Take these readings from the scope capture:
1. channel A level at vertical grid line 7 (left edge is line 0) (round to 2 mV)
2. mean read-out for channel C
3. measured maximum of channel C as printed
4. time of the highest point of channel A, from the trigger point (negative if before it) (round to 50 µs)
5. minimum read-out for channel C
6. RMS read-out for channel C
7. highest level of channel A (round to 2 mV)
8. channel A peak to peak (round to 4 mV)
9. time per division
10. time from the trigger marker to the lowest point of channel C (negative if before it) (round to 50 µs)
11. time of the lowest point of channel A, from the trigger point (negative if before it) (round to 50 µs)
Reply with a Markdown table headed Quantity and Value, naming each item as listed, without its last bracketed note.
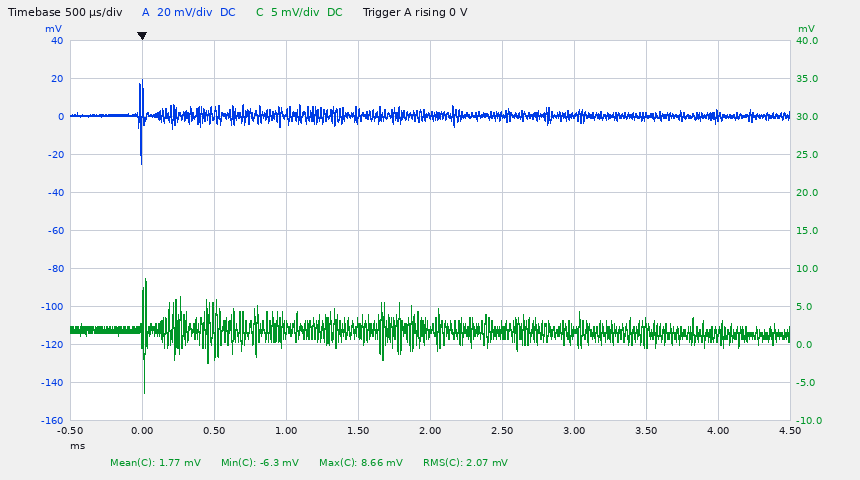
| Quantity | Value |
|---|---|
| channel A level at vertical grid line 7 (left edge is line 0) | 0 mV |
| mean read-out for channel C | 1.77 mV |
| measured maximum of channel C as printed | 8.66 mV |
| time of the highest point of channel A, from the trigger point (negative if before it) | 0 µs |
| minimum read-out for channel C | -6.3 mV |
| RMS read-out for channel C | 2.07 mV |
| highest level of channel A | 20 mV |
| channel A peak to peak | 44 mV |
| time per division | 500 µs |
| time from the trigger marker to the lowest point of channel C (negative if before it) | 0 µs |
| time of the lowest point of channel A, from the trigger point (negative if before it) | 0 µs |
